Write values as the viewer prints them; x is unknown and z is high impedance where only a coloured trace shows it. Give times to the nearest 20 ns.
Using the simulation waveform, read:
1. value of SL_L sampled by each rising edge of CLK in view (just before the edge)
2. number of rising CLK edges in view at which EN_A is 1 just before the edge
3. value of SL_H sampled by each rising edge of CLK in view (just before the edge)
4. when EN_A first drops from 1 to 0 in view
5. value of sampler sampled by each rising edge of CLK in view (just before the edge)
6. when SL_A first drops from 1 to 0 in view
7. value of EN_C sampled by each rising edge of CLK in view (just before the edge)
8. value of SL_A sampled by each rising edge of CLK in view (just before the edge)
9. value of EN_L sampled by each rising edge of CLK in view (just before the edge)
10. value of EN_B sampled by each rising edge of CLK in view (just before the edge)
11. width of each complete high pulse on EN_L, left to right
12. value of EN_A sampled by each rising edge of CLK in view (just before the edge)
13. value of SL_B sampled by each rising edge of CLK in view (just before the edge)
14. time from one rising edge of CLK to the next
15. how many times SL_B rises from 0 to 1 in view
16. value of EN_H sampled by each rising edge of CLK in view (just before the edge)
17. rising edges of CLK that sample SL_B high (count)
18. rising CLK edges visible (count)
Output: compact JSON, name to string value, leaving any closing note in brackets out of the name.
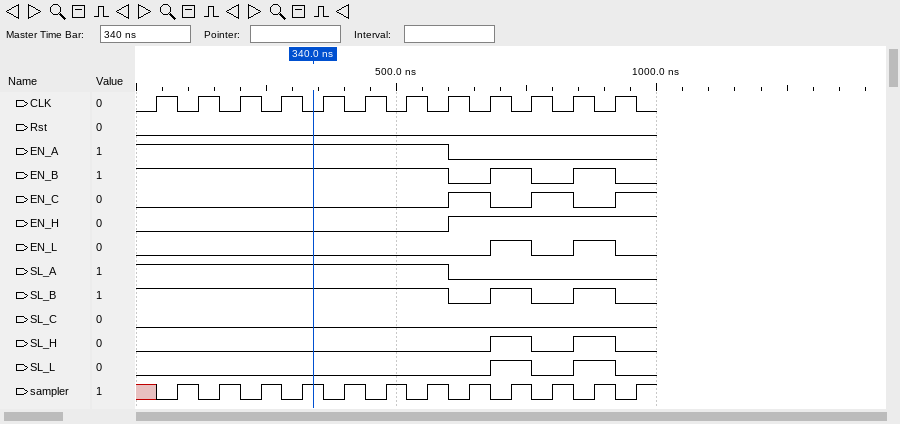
{"value of SL_L sampled by each rising edge of CLK in view": "0 0 0 0 0 0 0 0 0 1 0 1", "number of rising CLK edges in view at which EN_A is 1 just before the edge": "8", "value of SL_H sampled by each rising edge of CLK in view": "0 0 0 0 0 0 0 0 0 1 0 1", "when EN_A first drops from 1 to 0 in view": "600 ns", "value of sampler sampled by each rising edge of CLK in view": "x 1 1 1 1 1 1 1 1 1 1 1", "when SL_A first drops from 1 to 0 in view": "600 ns", "value of EN_C sampled by each rising edge of CLK in view": "0 0 0 0 0 0 0 0 1 0 1 0", "value of SL_A sampled by each rising edge of CLK in view": "1 1 1 1 1 1 1 1 0 0 0 0", "value of EN_L sampled by each rising edge of CLK in view": "0 0 0 0 0 0 0 0 0 1 0 1", "value of EN_B sampled by each rising edge of CLK in view": "1 1 1 1 1 1 1 1 0 1 0 1", "width of each complete high pulse on EN_L, left to right": "80 ns, 80 ns", "value of EN_A sampled by each rising edge of CLK in view": "1 1 1 1 1 1 1 1 0 0 0 0", "value of SL_B sampled by each rising edge of CLK in view": "1 1 1 1 1 1 1 1 0 1 0 1", "time from one rising edge of CLK to the next": "80 ns", "how many times SL_B rises from 0 to 1 in view": "2", "value of EN_H sampled by each rising edge of CLK in view": "0 0 0 0 0 0 0 0 1 1 1 1", "rising edges of CLK that sample SL_B high": "10", "rising CLK edges visible": "12"}
